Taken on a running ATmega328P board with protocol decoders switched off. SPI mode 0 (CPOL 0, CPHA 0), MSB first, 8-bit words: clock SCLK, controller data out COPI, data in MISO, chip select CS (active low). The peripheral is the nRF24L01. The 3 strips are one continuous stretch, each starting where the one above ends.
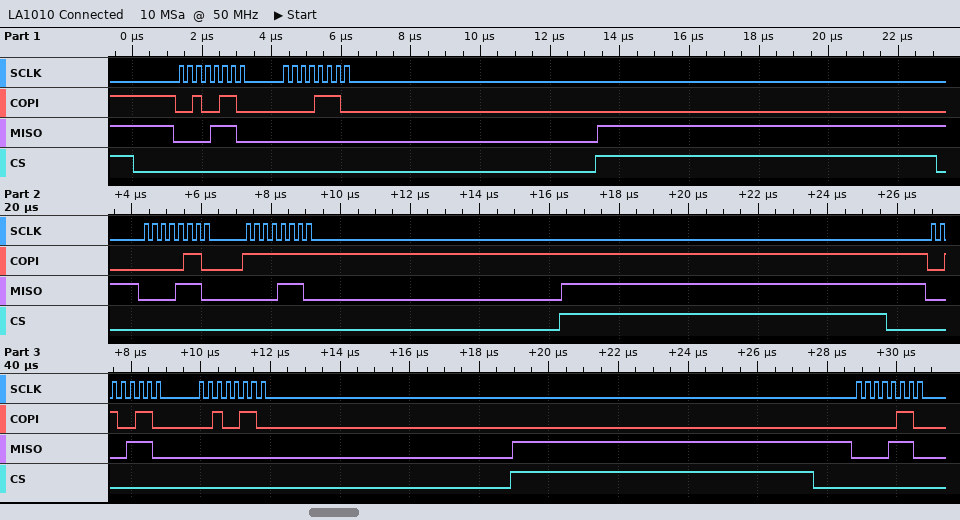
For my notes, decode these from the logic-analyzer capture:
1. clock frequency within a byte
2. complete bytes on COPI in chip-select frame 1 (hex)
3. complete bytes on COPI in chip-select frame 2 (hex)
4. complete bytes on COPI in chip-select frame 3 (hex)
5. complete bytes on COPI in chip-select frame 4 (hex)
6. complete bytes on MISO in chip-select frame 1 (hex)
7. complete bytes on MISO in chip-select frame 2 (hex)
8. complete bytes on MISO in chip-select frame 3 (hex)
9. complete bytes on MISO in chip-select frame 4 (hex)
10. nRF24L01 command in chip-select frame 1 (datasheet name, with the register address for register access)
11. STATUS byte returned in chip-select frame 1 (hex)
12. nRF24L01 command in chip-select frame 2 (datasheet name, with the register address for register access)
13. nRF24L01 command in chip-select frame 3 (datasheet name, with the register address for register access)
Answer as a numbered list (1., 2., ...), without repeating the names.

1. 4 MHz
2. 26 0E
3. 06 FF
4. 26 26
5. 06
6. 0E 00
7. 0E 0E
8. 0E 00
9. 0E
10. W_REGISTER 0x06
11. 0x0E
12. R_REGISTER 0x06
13. W_REGISTER 0x06
